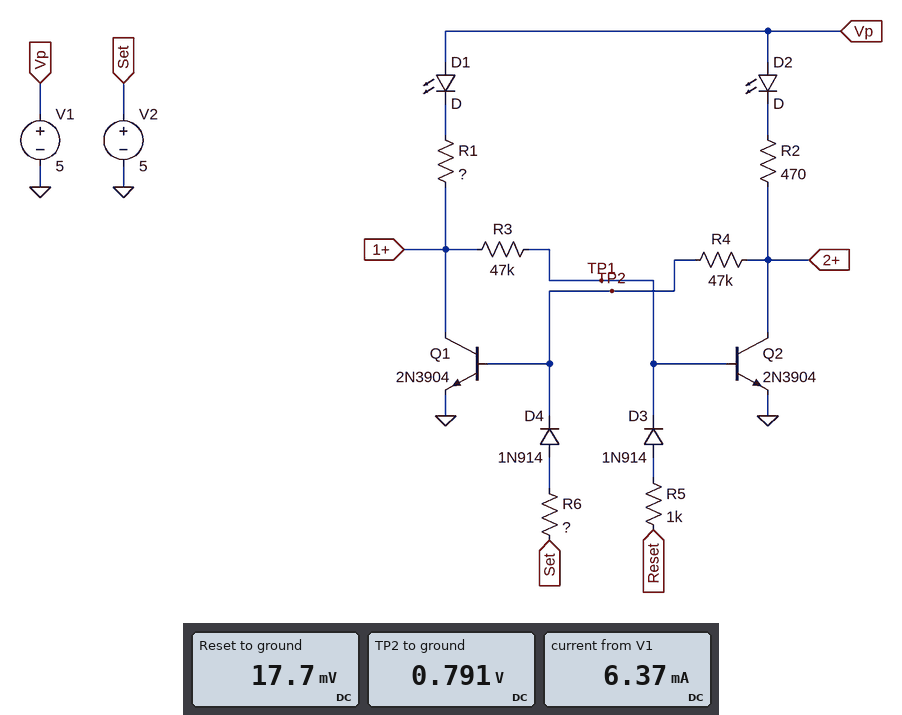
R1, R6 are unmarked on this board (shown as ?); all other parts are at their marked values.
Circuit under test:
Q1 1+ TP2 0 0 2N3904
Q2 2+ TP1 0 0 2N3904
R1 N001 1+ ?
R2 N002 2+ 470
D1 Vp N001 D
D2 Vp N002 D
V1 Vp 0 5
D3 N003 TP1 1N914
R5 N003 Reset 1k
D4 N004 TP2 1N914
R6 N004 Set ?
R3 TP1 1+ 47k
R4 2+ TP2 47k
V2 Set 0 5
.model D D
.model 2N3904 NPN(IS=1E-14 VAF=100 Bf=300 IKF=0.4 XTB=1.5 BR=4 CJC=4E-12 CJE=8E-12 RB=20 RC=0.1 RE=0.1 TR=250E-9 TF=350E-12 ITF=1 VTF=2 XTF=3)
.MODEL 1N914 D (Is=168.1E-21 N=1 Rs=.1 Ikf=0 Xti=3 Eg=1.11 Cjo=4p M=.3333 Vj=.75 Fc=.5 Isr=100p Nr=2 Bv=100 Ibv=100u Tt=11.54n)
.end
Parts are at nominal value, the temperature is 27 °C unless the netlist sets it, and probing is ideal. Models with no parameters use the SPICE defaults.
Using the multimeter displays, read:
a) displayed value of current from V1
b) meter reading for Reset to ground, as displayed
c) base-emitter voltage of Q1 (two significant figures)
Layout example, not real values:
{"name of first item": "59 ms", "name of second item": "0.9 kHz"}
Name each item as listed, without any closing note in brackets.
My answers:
{"displayed value of current from V1": "6.37 mA", "meter reading for Reset to ground, as displayed": "17.7 mV", "base-emitter voltage of Q1": "790 mV"}
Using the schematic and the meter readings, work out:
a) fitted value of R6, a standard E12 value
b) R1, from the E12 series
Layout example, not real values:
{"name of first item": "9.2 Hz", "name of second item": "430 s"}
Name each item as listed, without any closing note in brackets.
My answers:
{"fitted value of R6, a standard E12 value": "1.2 kΩ", "R1, from the E12 series": "680 Ω"}
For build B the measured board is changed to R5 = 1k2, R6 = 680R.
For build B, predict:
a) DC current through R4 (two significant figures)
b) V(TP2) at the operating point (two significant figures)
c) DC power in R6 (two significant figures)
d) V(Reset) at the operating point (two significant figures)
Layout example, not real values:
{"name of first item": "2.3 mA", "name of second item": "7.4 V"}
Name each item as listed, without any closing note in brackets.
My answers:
{"DC current through R4": "75 µA", "V(TP2) at the operating point": "840 mV", "DC power in R6": "15 mW", "V(Reset) at the operating point": "14 mV"}
